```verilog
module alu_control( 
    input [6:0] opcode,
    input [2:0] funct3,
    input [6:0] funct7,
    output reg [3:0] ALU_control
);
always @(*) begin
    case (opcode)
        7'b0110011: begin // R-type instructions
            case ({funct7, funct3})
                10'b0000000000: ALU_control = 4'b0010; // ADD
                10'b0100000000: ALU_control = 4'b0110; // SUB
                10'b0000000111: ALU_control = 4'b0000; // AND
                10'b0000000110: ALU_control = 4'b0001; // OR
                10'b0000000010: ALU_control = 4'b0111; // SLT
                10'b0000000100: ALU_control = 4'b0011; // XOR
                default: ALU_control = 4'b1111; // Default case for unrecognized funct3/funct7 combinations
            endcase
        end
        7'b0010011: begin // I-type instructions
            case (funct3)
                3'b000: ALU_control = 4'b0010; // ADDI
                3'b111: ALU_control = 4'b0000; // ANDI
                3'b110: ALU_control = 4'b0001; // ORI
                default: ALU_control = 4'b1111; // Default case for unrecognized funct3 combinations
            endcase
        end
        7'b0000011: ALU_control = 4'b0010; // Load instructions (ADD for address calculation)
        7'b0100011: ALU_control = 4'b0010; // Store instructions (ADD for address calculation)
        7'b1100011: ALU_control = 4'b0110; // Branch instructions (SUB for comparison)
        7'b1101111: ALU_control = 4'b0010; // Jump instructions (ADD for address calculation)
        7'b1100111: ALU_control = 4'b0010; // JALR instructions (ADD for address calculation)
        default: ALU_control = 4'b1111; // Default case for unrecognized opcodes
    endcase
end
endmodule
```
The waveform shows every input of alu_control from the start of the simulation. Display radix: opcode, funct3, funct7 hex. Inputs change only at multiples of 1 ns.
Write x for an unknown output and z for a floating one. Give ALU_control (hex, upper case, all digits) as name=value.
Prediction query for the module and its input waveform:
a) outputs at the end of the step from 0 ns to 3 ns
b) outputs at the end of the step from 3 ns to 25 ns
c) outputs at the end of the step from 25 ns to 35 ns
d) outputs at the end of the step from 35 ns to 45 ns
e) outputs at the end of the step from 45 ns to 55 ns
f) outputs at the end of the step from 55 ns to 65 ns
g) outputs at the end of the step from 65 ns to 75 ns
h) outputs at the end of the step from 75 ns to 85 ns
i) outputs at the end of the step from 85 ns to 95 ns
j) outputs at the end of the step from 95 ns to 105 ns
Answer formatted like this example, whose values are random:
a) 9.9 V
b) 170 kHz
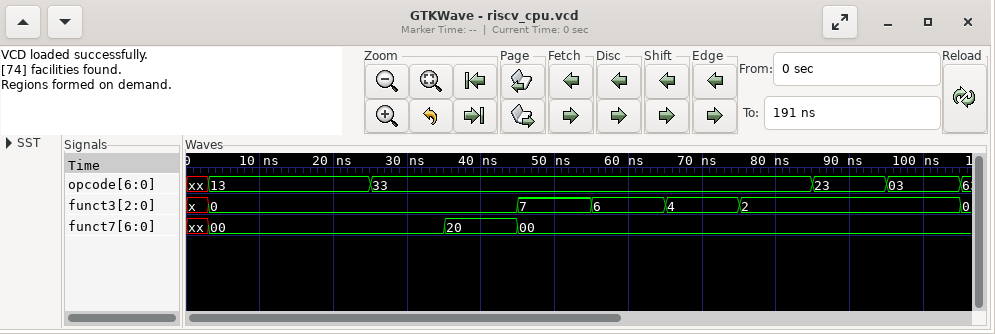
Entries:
a) ALU_control=x
b) ALU_control=2
c) ALU_control=2
d) ALU_control=6
e) ALU_control=0
f) ALU_control=1
g) ALU_control=3
h) ALU_control=7
i) ALU_control=2
j) ALU_control=2
